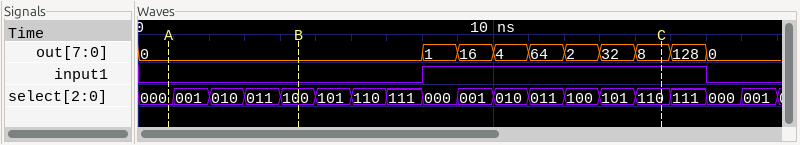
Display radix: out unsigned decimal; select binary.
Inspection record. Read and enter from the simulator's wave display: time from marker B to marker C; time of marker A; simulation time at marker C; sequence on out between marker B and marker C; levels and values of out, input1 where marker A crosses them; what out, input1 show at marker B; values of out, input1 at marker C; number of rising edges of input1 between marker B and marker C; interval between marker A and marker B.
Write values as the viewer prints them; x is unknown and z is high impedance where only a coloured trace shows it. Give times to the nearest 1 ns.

10 ns
1 ns
15 ns
0, 1, 16, 4, 64, 2, 32, 8
out=0, input1=0
out=0, input1=0
out=8, input1=1
1
4 ns
